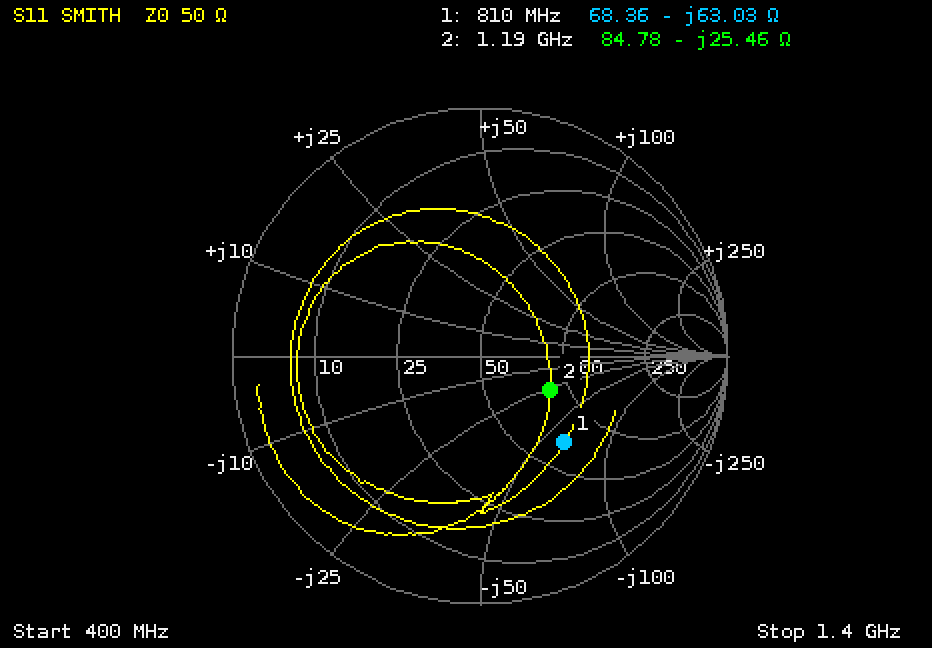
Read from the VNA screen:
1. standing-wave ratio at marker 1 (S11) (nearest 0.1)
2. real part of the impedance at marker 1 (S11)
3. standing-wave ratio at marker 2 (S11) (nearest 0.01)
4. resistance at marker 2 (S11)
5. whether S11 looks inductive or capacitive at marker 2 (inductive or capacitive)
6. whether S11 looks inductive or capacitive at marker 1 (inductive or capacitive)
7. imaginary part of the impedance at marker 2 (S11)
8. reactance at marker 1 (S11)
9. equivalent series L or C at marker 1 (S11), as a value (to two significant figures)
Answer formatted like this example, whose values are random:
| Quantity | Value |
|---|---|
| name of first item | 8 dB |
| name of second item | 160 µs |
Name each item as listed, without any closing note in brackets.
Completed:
| Quantity | Value |
|---|---|
| standing-wave ratio at marker 1 (S11) | 2.9 |
| real part of the impedance at marker 1 | 68.36 Ω |
| standing-wave ratio at marker 2 (S11) | 1.92 |
| resistance at marker 2 | 84.78 Ω |
| whether S11 looks inductive or capacitive at marker 2 | capacitive |
| whether S11 looks inductive or capacitive at marker 1 | capacitive |
| imaginary part of the impedance at marker 2 | -25.46 Ω |
| reactance at marker 1 | -63.03 Ω |
| equivalent series L or C at marker 1 (S11), as a value | 3.1 pF |
